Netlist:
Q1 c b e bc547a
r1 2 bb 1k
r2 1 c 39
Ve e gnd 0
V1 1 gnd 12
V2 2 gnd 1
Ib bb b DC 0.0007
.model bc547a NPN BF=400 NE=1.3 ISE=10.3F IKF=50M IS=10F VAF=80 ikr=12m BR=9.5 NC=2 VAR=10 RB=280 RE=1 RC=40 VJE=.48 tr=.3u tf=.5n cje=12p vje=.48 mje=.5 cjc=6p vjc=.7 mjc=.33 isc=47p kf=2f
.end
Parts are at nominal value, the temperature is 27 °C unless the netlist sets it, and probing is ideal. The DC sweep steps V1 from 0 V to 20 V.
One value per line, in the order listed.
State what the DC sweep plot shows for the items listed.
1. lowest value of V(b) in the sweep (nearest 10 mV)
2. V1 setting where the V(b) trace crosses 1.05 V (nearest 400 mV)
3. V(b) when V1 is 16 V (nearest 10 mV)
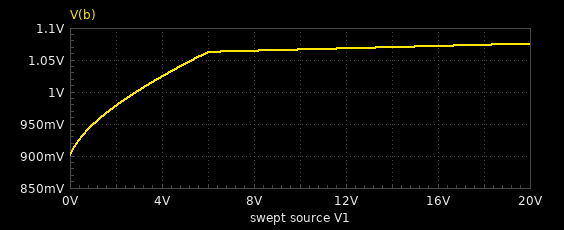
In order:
900 mV
5.2 V
1.07 V
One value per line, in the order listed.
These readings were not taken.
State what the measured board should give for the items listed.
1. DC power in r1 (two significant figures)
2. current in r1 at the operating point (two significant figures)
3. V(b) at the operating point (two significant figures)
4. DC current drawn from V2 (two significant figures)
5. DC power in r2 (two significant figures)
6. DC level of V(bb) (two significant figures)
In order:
490 µW
700 µA
1.1 V
700 µA
240 mW
300 mV
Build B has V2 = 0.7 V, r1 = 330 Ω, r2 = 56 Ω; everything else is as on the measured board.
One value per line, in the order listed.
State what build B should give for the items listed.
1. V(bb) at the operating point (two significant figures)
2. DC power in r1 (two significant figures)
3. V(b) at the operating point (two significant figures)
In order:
470 mV
160 µW
1.1 V
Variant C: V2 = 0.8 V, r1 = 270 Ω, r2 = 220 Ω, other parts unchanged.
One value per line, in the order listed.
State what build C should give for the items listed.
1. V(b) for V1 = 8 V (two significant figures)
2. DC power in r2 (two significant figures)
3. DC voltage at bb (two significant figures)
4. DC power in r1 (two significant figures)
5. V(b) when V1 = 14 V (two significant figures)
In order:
990 mV
460 mW
610 mV
130 µW
1.0 V
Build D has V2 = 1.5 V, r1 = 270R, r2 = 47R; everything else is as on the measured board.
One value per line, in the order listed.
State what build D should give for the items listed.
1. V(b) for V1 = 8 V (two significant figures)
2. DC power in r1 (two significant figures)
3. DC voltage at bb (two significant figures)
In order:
1.1 V
130 µW
1.3 V
